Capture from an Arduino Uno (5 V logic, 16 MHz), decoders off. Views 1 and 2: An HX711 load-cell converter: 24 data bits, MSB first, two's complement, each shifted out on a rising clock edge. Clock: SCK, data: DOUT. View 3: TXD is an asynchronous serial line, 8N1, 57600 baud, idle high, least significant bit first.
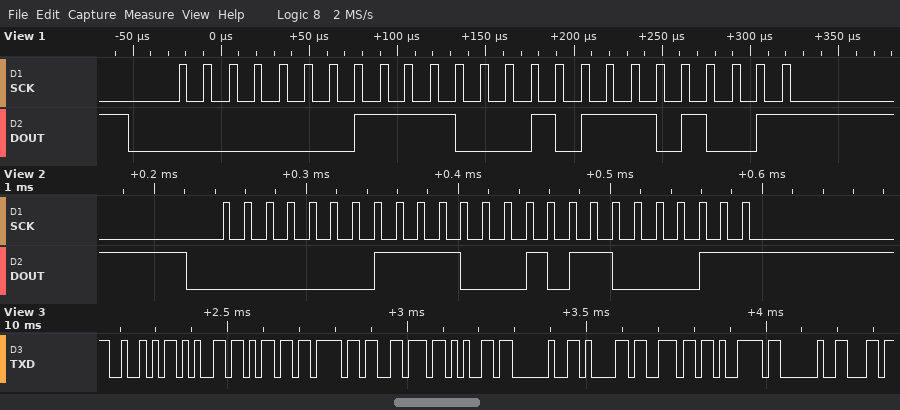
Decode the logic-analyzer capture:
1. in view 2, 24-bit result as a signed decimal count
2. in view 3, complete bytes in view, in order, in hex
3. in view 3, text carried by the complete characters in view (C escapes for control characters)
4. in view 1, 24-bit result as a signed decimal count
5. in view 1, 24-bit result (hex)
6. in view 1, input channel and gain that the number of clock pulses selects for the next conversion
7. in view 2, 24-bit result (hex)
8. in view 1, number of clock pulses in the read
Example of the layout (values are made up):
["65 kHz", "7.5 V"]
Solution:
["123587", "52 65 6D 6F 76 65 20 61 6E 79 20", "\"Remove any \"", "123625", "0x01E2E9", "channel A, gain 128", "0x01E2C3", "25"]
